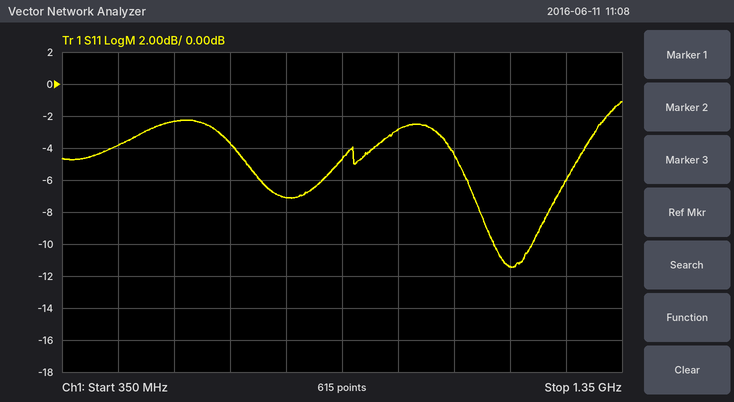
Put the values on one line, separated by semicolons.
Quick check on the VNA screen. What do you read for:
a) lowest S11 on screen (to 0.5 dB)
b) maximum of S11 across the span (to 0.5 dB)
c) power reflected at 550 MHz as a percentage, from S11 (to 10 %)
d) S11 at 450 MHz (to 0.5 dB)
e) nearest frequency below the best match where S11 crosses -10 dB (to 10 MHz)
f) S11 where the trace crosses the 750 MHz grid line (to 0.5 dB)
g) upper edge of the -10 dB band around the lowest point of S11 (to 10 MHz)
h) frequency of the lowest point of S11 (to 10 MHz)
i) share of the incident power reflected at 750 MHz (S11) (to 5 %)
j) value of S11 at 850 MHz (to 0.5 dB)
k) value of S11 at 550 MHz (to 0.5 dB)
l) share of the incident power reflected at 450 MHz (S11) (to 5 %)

-11.5 dB; -1.0 dB; 60 %; -4.0 dB; 1.12 GHz; -7.0 dB; 1.19 GHz; 1.15 GHz; 20 %; -4.5 dB; -2.5 dB; 40 %
